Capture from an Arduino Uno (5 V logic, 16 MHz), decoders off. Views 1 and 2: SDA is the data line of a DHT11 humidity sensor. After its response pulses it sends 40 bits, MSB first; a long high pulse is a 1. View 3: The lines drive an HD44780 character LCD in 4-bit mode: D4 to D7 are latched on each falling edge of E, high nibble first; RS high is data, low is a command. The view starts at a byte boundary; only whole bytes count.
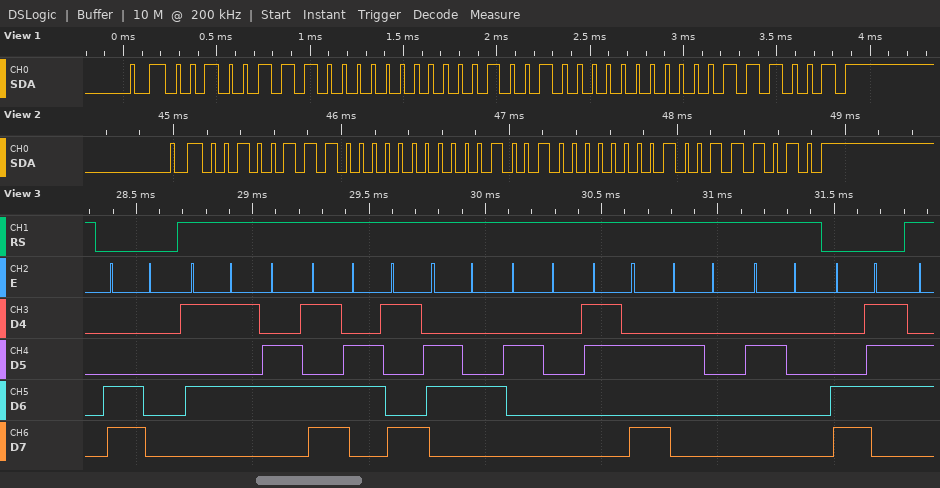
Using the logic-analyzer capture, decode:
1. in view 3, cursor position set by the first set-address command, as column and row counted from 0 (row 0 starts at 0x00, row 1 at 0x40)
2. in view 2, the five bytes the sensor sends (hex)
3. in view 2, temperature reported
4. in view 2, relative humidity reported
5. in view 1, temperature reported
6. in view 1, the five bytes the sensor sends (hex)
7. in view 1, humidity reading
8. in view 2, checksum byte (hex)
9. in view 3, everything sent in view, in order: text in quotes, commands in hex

column 0, row 1
27 00 12 01 3A
18.1 °C
39 %
18.0 °C
27 00 12 00 39
39 %
0x3A
0xC0 "Umid :  " 0xC7
